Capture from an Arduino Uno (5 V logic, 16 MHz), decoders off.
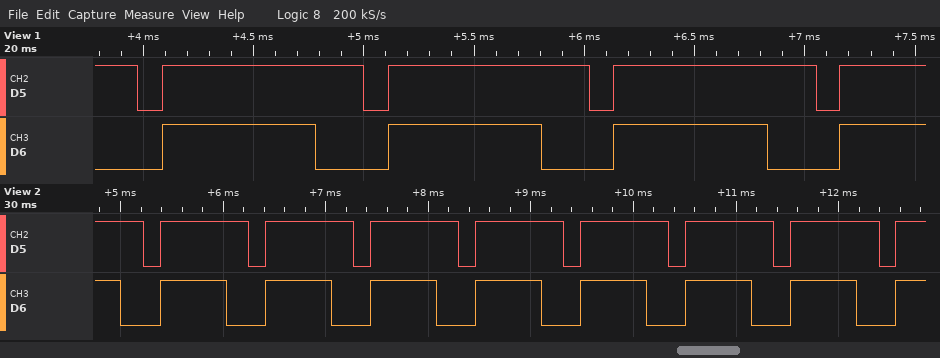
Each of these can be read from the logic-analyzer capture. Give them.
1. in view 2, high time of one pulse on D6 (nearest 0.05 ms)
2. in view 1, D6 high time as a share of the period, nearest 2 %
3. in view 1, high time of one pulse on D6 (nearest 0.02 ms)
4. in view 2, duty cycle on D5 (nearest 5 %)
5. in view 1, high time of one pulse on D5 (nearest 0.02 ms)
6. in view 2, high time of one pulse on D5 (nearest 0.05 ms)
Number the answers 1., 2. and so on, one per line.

1. 0.65 ms
2. 68 %
3. 0.70 ms
4. 85 %
5. 0.92 ms
6. 0.85 ms
